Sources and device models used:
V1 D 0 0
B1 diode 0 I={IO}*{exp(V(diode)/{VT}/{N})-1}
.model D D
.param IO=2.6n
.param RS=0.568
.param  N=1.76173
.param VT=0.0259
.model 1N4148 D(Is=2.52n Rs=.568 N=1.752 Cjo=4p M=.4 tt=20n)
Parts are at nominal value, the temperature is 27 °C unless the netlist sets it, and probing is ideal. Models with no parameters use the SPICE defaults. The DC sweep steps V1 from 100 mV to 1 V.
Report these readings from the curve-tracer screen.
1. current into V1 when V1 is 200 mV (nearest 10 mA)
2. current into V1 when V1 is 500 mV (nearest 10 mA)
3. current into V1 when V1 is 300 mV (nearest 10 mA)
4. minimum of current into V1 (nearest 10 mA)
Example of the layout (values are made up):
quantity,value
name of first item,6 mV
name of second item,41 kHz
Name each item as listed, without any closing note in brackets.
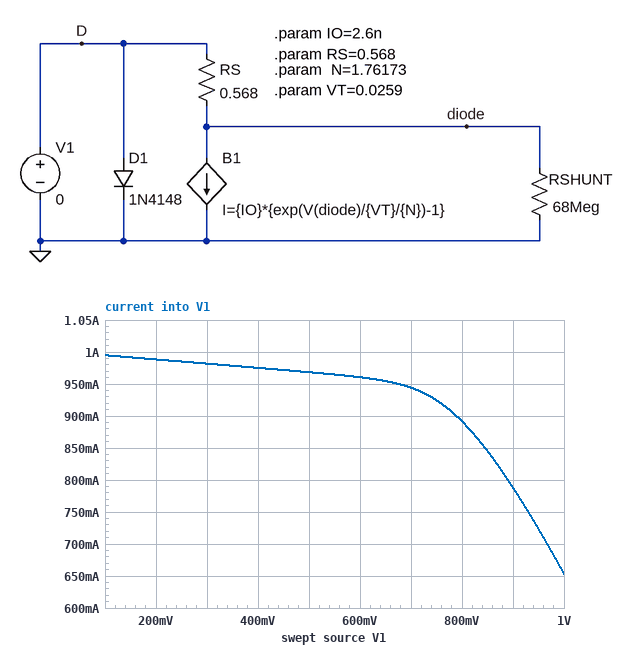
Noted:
quantity,value
current into V1 when V1 is 200 mV,990 mA
current into V1 when V1 is 500 mV,970 mA
current into V1 when V1 is 300 mV,980 mA
minimum of current into V1,650 mA
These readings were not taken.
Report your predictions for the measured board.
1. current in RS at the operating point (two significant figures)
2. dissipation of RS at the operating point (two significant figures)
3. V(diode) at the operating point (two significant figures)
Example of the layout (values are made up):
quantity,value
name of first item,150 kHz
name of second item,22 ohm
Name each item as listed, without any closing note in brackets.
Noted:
quantity,value
current in RS at the operating point,1.0 A
dissipation of RS at the operating point,570 mW
V(diode) at the operating point,570 mV
